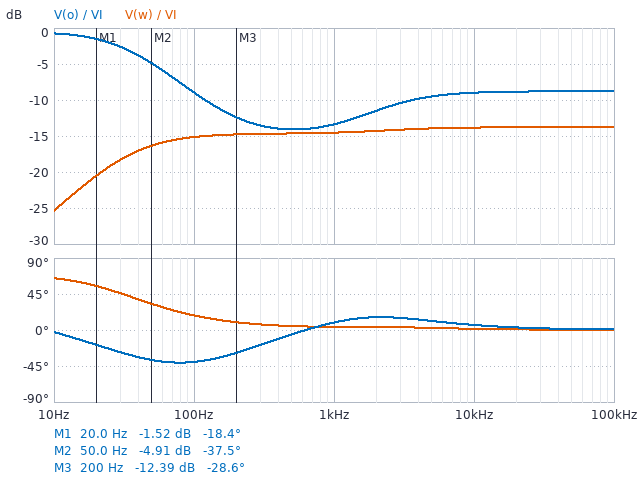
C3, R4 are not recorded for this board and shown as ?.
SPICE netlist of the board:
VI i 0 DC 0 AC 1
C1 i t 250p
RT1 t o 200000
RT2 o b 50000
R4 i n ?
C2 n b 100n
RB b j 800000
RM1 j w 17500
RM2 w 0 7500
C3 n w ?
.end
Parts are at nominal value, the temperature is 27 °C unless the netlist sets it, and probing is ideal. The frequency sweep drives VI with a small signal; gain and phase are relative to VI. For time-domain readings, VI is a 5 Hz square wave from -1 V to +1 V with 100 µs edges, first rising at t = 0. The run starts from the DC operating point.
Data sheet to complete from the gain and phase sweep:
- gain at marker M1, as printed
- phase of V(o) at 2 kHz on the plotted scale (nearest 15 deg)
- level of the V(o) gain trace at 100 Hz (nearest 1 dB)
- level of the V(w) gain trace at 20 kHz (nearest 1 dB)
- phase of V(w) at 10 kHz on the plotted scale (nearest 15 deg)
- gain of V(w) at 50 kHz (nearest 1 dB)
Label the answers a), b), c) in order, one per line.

a) -1.52 dB
b) 15 deg
c) -9 dB
d) -14 dB
e) 0 deg
f) -14 dB
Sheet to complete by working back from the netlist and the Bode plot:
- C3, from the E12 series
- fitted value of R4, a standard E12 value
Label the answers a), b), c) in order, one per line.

a) 120 nF
b) 33 kΩ
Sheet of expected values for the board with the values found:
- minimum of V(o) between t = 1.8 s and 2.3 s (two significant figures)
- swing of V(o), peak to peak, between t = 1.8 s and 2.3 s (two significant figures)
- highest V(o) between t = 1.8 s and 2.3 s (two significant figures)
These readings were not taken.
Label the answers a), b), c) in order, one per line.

a) -1.2 V
b) 2.5 V
c) 1.2 V
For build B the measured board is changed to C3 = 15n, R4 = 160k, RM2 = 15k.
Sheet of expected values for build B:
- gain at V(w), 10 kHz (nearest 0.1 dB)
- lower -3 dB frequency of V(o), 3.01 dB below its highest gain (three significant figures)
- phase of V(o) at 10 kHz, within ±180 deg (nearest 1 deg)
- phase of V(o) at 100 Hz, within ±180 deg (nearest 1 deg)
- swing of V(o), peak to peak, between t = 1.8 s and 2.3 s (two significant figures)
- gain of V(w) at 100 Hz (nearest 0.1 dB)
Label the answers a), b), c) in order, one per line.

a) -17.7 dB
b) 1.53 Hz
c) 8 deg
d) -43 deg
e) 2.2 V
f) -23.2 dB
